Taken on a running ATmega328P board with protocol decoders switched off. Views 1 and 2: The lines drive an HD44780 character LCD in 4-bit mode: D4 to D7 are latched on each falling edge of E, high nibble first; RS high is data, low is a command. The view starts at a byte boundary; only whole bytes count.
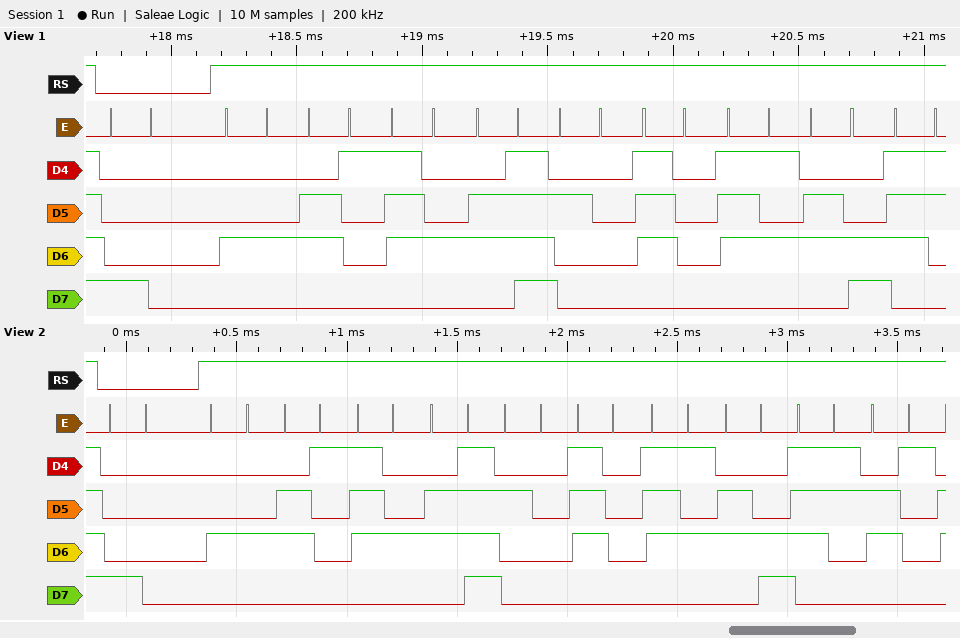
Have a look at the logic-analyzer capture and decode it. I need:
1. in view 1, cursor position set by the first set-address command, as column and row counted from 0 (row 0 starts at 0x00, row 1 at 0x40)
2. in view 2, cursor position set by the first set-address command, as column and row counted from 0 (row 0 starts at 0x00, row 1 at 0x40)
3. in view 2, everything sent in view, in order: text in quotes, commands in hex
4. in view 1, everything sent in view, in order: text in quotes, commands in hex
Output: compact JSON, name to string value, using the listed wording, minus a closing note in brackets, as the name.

{"in view 1, cursor position set by the first set-address command, as column and row counted from 0": "column 0, row 0", "in view 2, cursor position set by the first set-address command, as column and row counted from 0": "column 0, row 0", "in view 2, everything sent in view, in order: text in quotes, commands in hex": "0x80 \"Dato pulsa\"", "in view 1, everything sent in view, in order: text in quotes, commands in hex": "0x80 \"Dato puls\""}
